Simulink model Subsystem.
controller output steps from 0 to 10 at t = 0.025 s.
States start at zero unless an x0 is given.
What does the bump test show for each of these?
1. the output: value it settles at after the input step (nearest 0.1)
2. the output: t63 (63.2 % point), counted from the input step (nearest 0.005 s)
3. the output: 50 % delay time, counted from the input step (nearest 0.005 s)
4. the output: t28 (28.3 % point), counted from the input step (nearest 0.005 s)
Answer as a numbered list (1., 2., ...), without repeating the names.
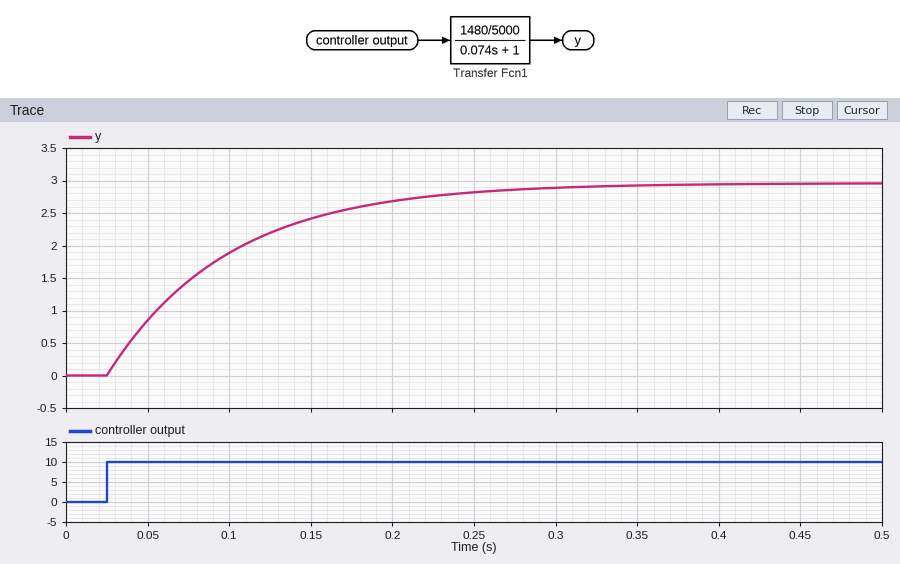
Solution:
1. 3.0
2. 0.075 s
3. 0.050 s
4. 0.025 s
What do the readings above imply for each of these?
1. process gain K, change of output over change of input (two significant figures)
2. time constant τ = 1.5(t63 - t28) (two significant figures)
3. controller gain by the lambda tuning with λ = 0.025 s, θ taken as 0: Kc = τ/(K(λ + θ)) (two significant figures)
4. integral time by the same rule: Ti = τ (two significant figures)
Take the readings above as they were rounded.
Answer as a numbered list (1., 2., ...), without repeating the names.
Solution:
1. 0.30
2. 0.075 s
3. 10
4. 0.075 s
